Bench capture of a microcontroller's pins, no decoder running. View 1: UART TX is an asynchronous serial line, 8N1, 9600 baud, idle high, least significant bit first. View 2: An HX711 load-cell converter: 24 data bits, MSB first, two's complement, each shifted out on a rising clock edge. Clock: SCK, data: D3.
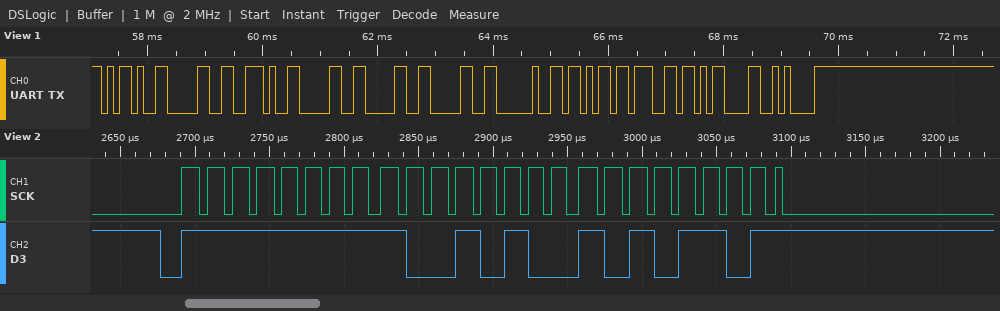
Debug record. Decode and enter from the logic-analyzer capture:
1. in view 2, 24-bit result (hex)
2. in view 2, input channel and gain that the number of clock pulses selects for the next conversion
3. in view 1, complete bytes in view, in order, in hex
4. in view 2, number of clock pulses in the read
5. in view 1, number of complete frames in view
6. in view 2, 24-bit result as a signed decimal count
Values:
0xFF94AD
channel A, gain 128
2D 30 2E 30 30 30 20 6B 67 0D 0A
25
11
-27475
